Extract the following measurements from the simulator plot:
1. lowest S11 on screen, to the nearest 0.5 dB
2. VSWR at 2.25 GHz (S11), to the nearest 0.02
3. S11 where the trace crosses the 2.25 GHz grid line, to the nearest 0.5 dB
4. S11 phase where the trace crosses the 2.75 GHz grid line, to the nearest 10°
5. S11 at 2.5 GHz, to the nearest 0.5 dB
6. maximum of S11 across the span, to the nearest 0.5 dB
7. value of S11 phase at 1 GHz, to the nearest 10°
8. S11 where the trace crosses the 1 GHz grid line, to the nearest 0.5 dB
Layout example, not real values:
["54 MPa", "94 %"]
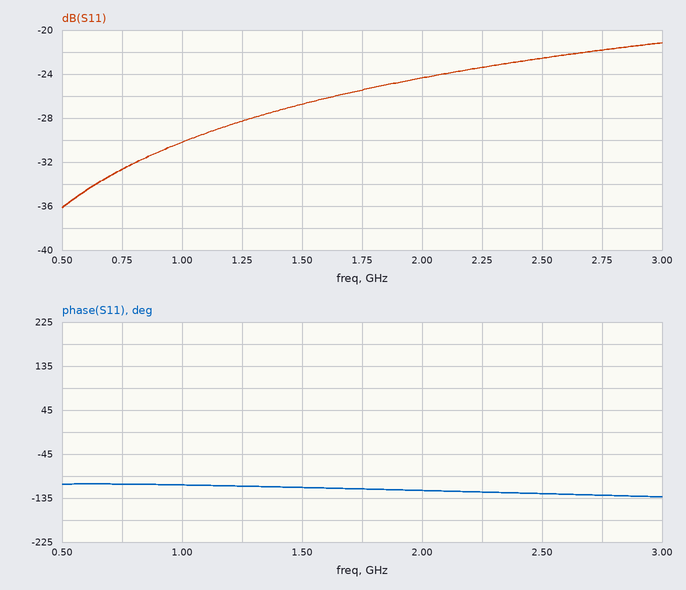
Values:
["-36.0 dB", "1.14", "-23.5 dB", "-130°", "-22.5 dB", "-21.0 dB", "-110°", "-30.0 dB"]
